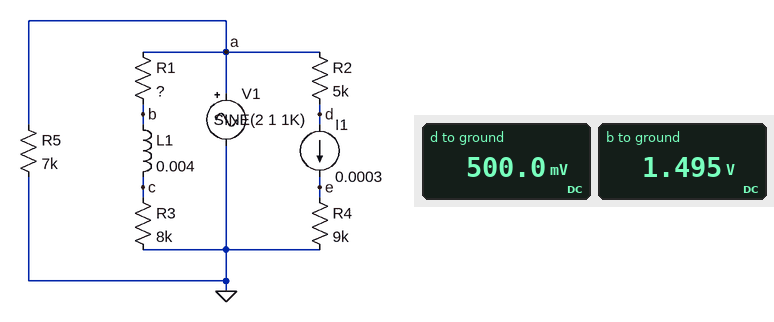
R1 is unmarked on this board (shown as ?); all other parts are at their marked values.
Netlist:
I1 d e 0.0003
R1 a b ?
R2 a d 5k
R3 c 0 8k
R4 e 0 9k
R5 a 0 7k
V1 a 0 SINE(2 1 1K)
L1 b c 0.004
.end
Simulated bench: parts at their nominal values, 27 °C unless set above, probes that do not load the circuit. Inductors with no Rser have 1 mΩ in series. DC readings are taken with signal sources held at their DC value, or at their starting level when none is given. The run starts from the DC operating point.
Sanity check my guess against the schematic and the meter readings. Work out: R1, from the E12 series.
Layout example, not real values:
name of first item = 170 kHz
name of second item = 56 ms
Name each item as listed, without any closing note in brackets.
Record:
R1, from the E12 series = 2.7 kΩ
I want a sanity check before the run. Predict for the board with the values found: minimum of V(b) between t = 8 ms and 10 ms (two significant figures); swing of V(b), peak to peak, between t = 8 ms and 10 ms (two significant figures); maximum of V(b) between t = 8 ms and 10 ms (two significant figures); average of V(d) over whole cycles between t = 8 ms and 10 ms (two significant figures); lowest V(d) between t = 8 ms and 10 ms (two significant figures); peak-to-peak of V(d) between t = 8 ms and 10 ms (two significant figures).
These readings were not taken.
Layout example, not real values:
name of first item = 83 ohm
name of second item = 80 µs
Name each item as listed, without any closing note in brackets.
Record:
minimum of V(b) between t = 8 ms and 10 ms = 750 mV
swing of V(b), peak to peak, between t = 8 ms and 10 ms = 1.5 V
maximum of V(b) between t = 8 ms and 10 ms = 2.2 V
average of V(d) over whole cycles between t = 8 ms and 10 ms = 500 mV
lowest V(d) between t = 8 ms and 10 ms = -500 mV
peak-to-peak of V(d) between t = 8 ms and 10 ms = 2.0 V
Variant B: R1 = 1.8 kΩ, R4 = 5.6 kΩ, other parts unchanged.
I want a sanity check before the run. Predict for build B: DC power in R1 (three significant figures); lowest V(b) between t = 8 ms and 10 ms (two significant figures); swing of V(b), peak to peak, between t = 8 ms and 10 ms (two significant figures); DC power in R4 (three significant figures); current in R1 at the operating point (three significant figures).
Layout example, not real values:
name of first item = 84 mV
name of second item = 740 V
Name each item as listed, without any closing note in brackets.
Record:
DC power in R1 = 75.0 µW
lowest V(b) between t = 8 ms and 10 ms = 820 mV
swing of V(b), peak to peak, between t = 8 ms and 10 ms = 1.6 V
DC power in R4 = 504 µW
current in R1 at the operating point = 204 µA
